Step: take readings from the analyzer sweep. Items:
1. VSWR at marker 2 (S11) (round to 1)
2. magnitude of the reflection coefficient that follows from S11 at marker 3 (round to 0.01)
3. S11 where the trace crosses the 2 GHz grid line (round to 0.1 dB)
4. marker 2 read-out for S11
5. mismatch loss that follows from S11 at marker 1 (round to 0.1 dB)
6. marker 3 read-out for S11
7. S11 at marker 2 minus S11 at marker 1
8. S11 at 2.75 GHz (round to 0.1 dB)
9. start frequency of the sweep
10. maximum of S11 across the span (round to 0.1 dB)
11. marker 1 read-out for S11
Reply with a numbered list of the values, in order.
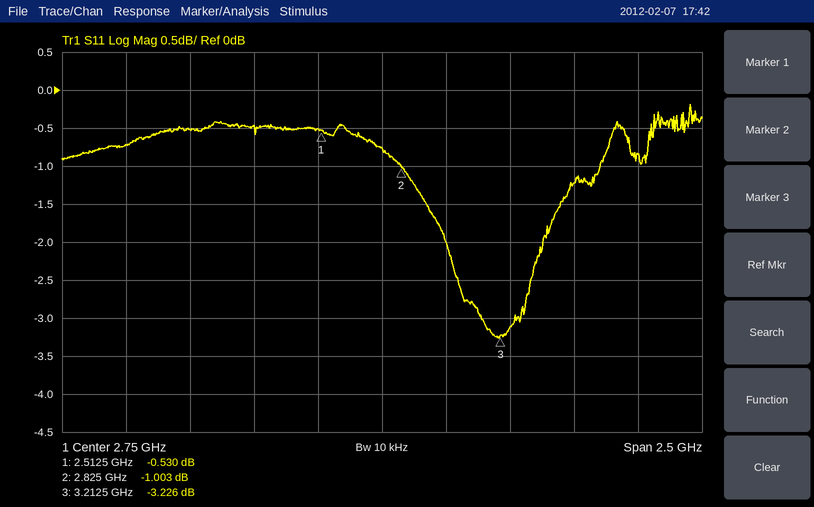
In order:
1. 17
2. 0.69
3. -0.5 dB
4. -1.003 dB
5. 9.4 dB
6. -3.226 dB
7. -0.473 dB
8. -0.8 dB
9. 1.5 GHz
10. -0.2 dB
11. -0.530 dB
